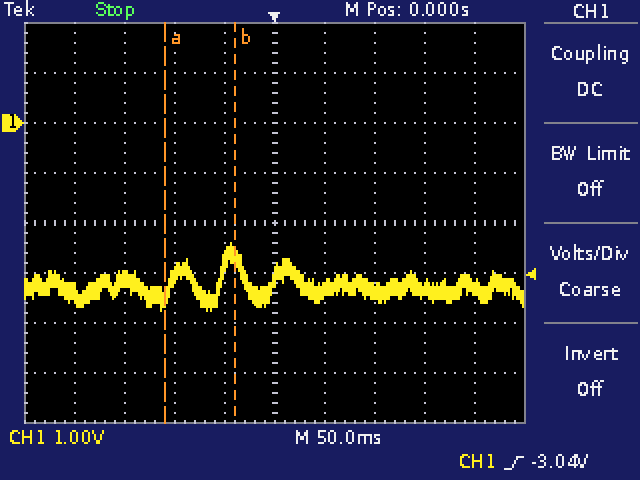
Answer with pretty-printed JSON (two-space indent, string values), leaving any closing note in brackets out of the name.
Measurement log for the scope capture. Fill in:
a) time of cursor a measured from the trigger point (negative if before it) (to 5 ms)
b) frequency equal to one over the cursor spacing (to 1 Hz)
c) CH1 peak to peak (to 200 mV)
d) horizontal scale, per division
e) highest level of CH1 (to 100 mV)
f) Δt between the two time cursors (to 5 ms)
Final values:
{
  "time of cursor a measured from the trigger point (negative if before it)": "-110 ms",
  "frequency equal to one over the cursor spacing": "14 Hz",
  "CH1 peak to peak": "1.4 V",
  "horizontal scale, per division": "50 ms",
  "highest level of CH1": "-2.4 V",
  "Δt between the two time cursors": "70 ms"
}
